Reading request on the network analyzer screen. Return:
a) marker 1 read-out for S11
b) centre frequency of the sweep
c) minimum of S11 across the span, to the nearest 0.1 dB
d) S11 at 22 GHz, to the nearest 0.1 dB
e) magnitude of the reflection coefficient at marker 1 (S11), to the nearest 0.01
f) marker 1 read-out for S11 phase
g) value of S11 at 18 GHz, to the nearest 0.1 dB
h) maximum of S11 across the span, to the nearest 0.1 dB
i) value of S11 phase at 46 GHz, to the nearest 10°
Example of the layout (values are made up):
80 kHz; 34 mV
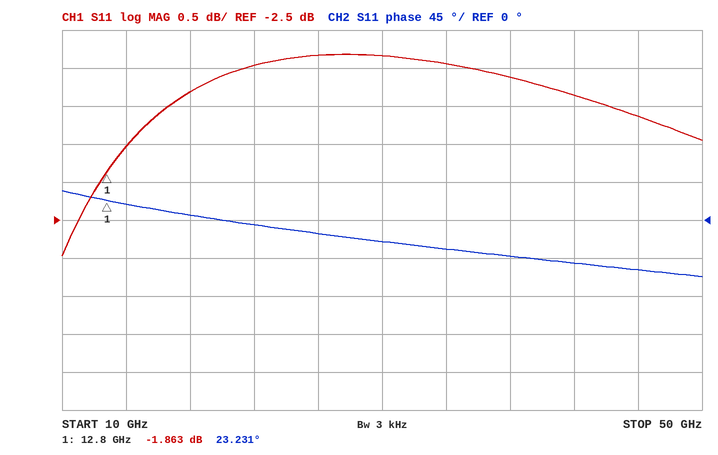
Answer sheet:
-1.863 dB; 30 GHz; -3.0 dB; -0.5 dB; 0.81; 23.231°; -0.8 dB; -0.3 dB; -60°
